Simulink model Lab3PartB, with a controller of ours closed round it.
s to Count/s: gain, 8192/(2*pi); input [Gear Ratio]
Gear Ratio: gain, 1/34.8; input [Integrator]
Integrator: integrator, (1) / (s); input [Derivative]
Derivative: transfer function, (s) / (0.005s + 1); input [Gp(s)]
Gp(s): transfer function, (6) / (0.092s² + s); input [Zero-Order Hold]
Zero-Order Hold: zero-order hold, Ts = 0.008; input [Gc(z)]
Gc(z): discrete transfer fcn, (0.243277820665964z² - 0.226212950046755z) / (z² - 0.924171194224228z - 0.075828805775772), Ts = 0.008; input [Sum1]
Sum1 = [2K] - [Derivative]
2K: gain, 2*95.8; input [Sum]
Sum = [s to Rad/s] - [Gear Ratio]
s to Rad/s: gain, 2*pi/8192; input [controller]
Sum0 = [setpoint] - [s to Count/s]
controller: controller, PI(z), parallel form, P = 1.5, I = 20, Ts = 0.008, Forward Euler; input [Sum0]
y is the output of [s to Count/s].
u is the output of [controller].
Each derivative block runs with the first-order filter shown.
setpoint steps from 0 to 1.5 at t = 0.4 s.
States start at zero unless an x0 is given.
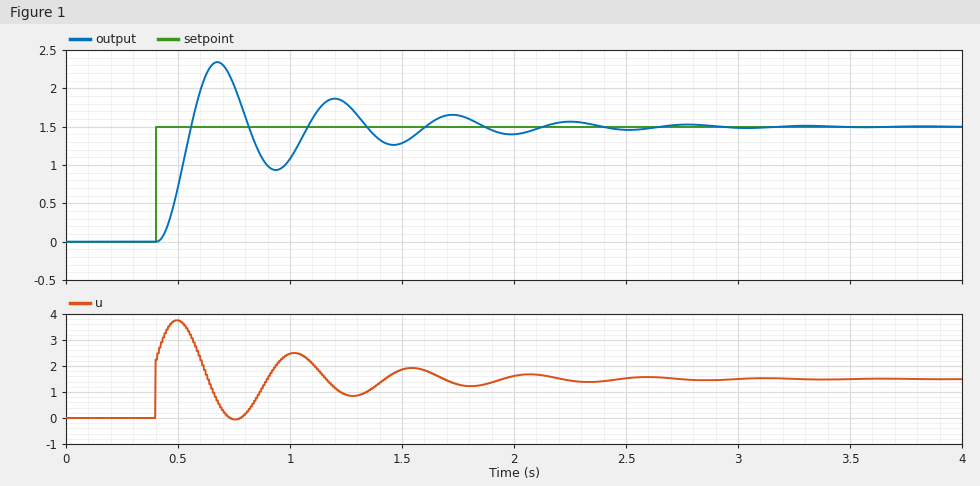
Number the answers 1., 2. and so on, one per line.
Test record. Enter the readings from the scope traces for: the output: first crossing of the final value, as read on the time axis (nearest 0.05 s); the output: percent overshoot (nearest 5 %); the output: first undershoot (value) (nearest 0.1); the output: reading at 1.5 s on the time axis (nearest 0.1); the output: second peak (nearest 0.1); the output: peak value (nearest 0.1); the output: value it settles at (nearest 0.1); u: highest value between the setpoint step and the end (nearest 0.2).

1. 0.55 s
2. 55 %
3. 0.9
4. 1.3
5. 1.9
6. 2.3
7. 1.5
8. 3.8
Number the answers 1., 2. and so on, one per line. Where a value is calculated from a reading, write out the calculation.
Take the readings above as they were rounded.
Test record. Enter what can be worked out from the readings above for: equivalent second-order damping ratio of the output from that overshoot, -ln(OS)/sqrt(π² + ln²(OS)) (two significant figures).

1. ln(0.55) = -0.598; 0.598 / sqrt(9.870 + 0.357) = 0.19
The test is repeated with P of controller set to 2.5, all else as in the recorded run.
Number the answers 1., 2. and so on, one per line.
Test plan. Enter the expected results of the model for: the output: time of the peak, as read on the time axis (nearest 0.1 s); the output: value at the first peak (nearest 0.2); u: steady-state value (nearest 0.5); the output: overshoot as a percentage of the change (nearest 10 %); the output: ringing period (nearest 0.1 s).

1. 0.6 s
2. 2.2
3. 1.5
4. 40 %
5. 0.4 s
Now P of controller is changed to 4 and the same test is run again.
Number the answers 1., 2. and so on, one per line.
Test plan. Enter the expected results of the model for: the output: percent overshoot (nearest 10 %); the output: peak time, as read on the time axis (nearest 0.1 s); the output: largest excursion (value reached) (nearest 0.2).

1. 40 %
2. 0.6 s
3. 2.2
